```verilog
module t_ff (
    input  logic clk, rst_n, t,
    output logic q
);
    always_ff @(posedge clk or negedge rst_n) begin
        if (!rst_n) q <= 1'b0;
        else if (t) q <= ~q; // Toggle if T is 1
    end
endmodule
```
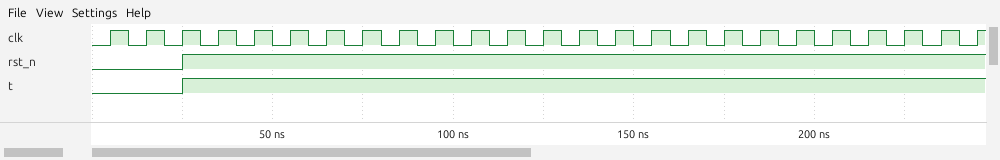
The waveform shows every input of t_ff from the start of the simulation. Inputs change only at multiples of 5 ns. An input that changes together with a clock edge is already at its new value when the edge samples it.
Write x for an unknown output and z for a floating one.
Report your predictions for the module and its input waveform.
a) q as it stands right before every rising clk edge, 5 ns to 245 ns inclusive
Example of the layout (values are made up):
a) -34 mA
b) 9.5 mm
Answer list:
a) 0 0 0 1 0 1 0 1 0 1 0 1 0 1 0 1 0 1 0 1 0 1 0 1 0
